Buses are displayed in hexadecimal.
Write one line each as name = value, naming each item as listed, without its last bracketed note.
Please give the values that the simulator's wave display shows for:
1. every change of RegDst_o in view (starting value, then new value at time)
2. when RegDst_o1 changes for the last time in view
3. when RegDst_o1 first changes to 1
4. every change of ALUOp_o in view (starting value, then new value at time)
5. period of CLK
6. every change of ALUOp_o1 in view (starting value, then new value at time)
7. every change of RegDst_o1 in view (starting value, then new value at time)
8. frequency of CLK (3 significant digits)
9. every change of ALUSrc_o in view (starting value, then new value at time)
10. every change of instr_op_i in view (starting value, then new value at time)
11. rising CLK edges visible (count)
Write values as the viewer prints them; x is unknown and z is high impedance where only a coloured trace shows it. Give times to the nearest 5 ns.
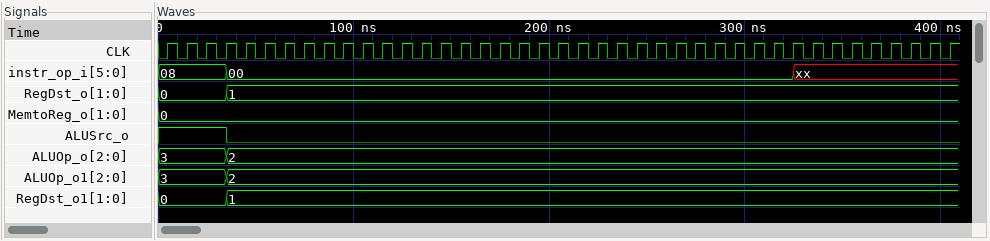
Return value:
every change of RegDst_o in view = 0, 1 at 35 ns
when RegDst_o1 changes for the last time in view = 35 ns
when RegDst_o1 first changes to 1 = 35 ns
every change of ALUOp_o in view = 3, 2 at 35 ns
period of CLK = 10 ns
every change of ALUOp_o1 in view = 3, 2 at 35 ns
every change of RegDst_o1 in view = 0, 1 at 35 ns
frequency of CLK = 100 MHz
every change of ALUSrc_o in view = 1, 0 at 35 ns
every change of instr_op_i in view = 08, 00 at 35 ns, xx at 325 ns
rising CLK edges visible = 41
